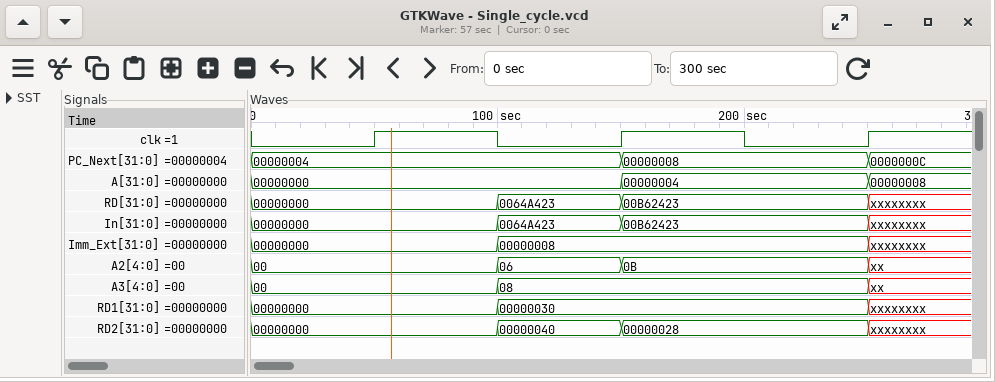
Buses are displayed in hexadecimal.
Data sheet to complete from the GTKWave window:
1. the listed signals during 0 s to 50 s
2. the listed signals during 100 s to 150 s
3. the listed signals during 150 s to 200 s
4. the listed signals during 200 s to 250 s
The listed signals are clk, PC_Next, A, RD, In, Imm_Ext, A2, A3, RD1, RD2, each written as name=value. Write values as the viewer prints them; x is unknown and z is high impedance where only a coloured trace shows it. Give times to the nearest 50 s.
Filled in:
clk=0, PC_Next=00000004, A=00000000, RD=00000000, In=00000000, Imm_Ext=00000000, A2=00, A3=00, RD1=00000000, RD2=00000000
clk=0, PC_Next=00000004, A=00000000, RD=0064A423, In=0064A423, Imm_Ext=00000008, A2=06, A3=08, RD1=00000030, RD2=00000040
clk=1, PC_Next=00000008, A=00000004, RD=00B62423, In=00B62423, Imm_Ext=00000008, A2=0B, A3=08, RD1=00000030, RD2=00000028
clk=0, PC_Next=00000008, A=00000004, RD=00B62423, In=00B62423, Imm_Ext=00000008, A2=0B, A3=08, RD1=00000030, RD2=00000028
